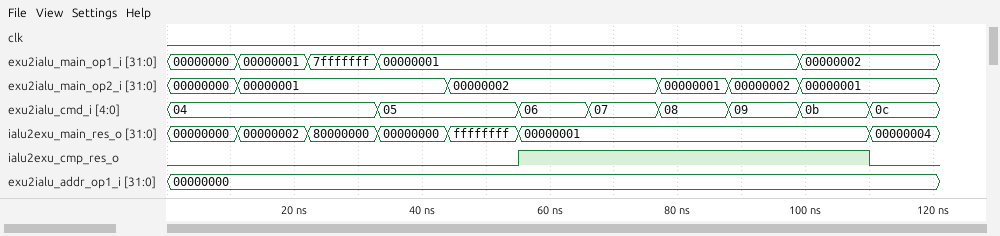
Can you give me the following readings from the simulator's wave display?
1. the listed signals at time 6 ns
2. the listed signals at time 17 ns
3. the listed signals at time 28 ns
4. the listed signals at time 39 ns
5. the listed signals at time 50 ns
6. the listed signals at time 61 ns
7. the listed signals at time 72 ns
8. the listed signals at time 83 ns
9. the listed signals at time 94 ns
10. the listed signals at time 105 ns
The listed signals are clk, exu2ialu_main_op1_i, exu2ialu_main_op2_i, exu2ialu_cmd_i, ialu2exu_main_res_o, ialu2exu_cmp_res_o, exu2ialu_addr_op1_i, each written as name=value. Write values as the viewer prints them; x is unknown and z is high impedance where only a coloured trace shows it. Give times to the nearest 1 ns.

clk=0, exu2ialu_main_op1_i=00000000, exu2ialu_main_op2_i=00000000, exu2ialu_cmd_i=04, ialu2exu_main_res_o=00000000, ialu2exu_cmp_res_o=0, exu2ialu_addr_op1_i=00000000
clk=0, exu2ialu_main_op1_i=00000001, exu2ialu_main_op2_i=00000001, exu2ialu_cmd_i=04, ialu2exu_main_res_o=00000002, ialu2exu_cmp_res_o=0, exu2ialu_addr_op1_i=00000000
clk=0, exu2ialu_main_op1_i=7fffffff, exu2ialu_main_op2_i=00000001, exu2ialu_cmd_i=04, ialu2exu_main_res_o=80000000, ialu2exu_cmp_res_o=0, exu2ialu_addr_op1_i=00000000
clk=0, exu2ialu_main_op1_i=00000001, exu2ialu_main_op2_i=00000001, exu2ialu_cmd_i=05, ialu2exu_main_res_o=00000000, ialu2exu_cmp_res_o=0, exu2ialu_addr_op1_i=00000000
clk=0, exu2ialu_main_op1_i=00000001, exu2ialu_main_op2_i=00000002, exu2ialu_cmd_i=05, ialu2exu_main_res_o=ffffffff, ialu2exu_cmp_res_o=0, exu2ialu_addr_op1_i=00000000
clk=0, exu2ialu_main_op1_i=00000001, exu2ialu_main_op2_i=00000002, exu2ialu_cmd_i=06, ialu2exu_main_res_o=00000001, ialu2exu_cmp_res_o=1, exu2ialu_addr_op1_i=00000000
clk=0, exu2ialu_main_op1_i=00000001, exu2ialu_main_op2_i=00000002, exu2ialu_cmd_i=07, ialu2exu_main_res_o=00000001, ialu2exu_cmp_res_o=1, exu2ialu_addr_op1_i=00000000
clk=0, exu2ialu_main_op1_i=00000001, exu2ialu_main_op2_i=00000001, exu2ialu_cmd_i=08, ialu2exu_main_res_o=00000001, ialu2exu_cmp_res_o=1, exu2ialu_addr_op1_i=00000000
clk=0, exu2ialu_main_op1_i=00000001, exu2ialu_main_op2_i=00000002, exu2ialu_cmd_i=09, ialu2exu_main_res_o=00000001, ialu2exu_cmp_res_o=1, exu2ialu_addr_op1_i=00000000
clk=0, exu2ialu_main_op1_i=00000002, exu2ialu_main_op2_i=00000001, exu2ialu_cmd_i=0b, ialu2exu_main_res_o=00000001, ialu2exu_cmp_res_o=1, exu2ialu_addr_op1_i=00000000
